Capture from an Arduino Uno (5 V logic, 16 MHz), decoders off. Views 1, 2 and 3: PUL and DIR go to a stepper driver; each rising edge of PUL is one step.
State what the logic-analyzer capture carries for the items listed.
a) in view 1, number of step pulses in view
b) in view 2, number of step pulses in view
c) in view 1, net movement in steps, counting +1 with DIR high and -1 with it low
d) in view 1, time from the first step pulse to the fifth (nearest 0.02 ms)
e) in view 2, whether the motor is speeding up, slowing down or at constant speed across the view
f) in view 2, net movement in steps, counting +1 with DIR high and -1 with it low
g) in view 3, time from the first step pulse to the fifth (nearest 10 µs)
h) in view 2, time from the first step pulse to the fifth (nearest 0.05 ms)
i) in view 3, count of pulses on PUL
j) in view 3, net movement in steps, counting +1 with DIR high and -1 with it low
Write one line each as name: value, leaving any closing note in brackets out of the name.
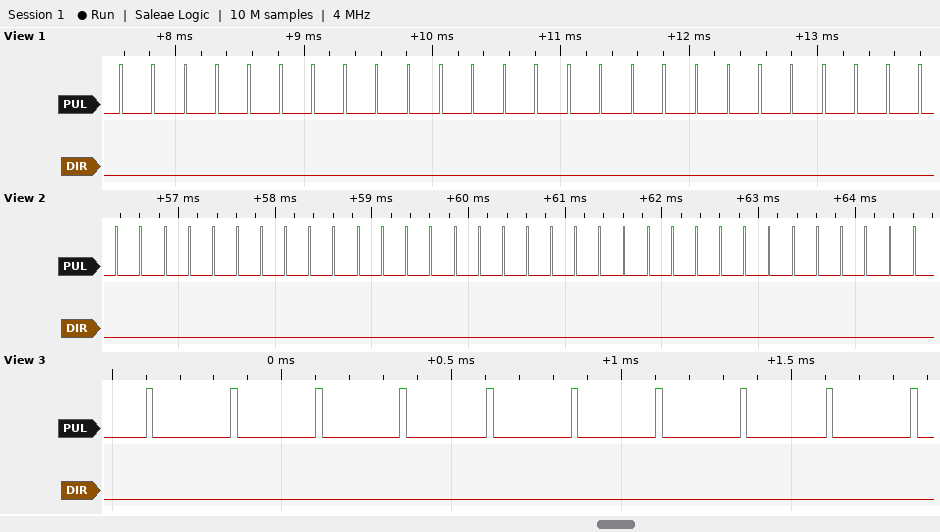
in view 1, number of step pulses in view: 26
in view 2, number of step pulses in view: 34
in view 1, net movement in steps, counting +1 with DIR high and -1 with it low: -26
in view 1, time from the first step pulse to the fifth: 1.00 ms
in view 2, whether the motor is speeding up, slowing down or at constant speed across the view: constant speed
in view 2, net movement in steps, counting +1 with DIR high and -1 with it low: -34
in view 3, time from the first step pulse to the fifth: 1000 µs
in view 2, time from the first step pulse to the fifth: 1.00 ms
in view 3, count of pulses on PUL: 10
in view 3, net movement in steps, counting +1 with DIR high and -1 with it low: -10
